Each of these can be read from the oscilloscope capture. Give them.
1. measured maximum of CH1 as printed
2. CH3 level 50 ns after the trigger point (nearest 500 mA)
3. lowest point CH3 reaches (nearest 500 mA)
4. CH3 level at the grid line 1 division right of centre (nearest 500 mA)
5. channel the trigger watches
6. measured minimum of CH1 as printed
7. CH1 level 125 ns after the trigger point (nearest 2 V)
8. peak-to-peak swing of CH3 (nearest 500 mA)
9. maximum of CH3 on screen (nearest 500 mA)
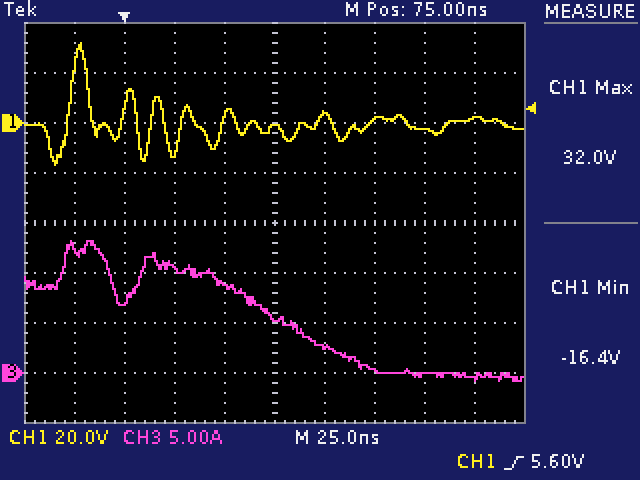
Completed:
32.0 V
9.0 A
-1.0 A
2.5 A
CH1
-16.4 V
2 V
14.0 A
13.0 A
